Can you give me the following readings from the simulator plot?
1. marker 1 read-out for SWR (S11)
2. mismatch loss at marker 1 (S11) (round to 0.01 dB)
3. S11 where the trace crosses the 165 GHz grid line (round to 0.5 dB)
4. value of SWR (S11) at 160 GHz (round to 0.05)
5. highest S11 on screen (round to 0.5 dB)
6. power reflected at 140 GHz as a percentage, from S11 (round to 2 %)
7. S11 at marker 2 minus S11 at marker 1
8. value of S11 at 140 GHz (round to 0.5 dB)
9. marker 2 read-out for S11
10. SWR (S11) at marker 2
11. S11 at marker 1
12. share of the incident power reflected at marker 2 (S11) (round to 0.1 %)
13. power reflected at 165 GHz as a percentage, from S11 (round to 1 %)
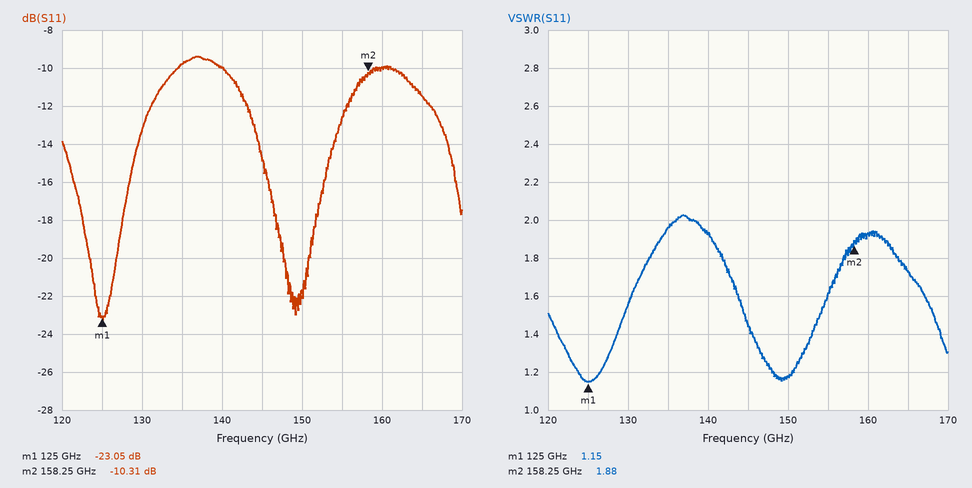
1.15
0.02 dB
-11.5 dB
1.95
-9.5 dB
10 %
12.74 dB
-10.0 dB
-10.31 dB
1.88
-23.05 dB
9.3 %
7 %
